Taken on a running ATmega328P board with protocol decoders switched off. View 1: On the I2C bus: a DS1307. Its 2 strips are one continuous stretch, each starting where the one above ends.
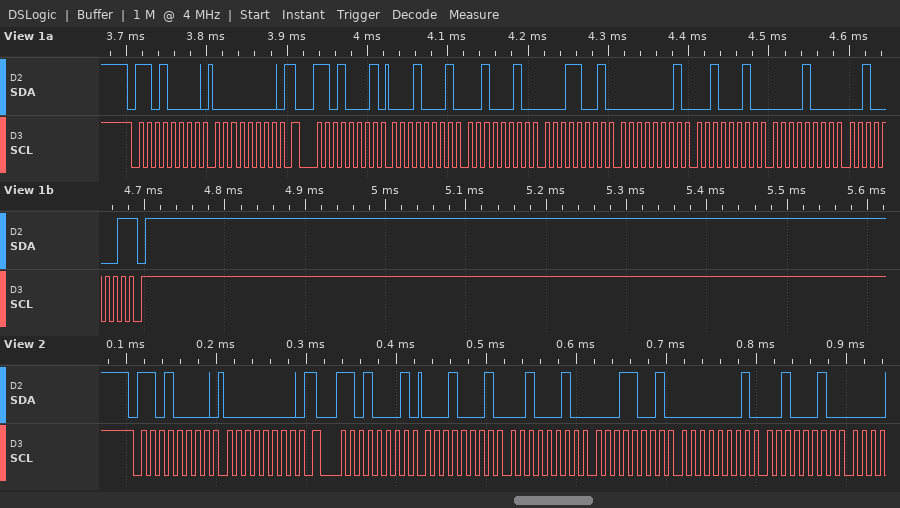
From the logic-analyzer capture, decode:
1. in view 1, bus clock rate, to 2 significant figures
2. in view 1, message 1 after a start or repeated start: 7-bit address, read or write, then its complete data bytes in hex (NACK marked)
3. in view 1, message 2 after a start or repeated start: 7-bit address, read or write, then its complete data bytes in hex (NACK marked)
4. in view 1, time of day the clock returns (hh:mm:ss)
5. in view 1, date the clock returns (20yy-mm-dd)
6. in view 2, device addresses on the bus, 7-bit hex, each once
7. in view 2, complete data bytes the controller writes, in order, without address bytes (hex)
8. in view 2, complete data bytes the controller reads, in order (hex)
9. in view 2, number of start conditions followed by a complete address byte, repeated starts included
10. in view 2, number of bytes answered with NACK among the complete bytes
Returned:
100 kHz
0x68 write: 00
0x68 read: 11 22 19 01 22 08 21 NACK
19:22:11
2021-08-22
0x68
00
11 22 19 01 22
2
0
